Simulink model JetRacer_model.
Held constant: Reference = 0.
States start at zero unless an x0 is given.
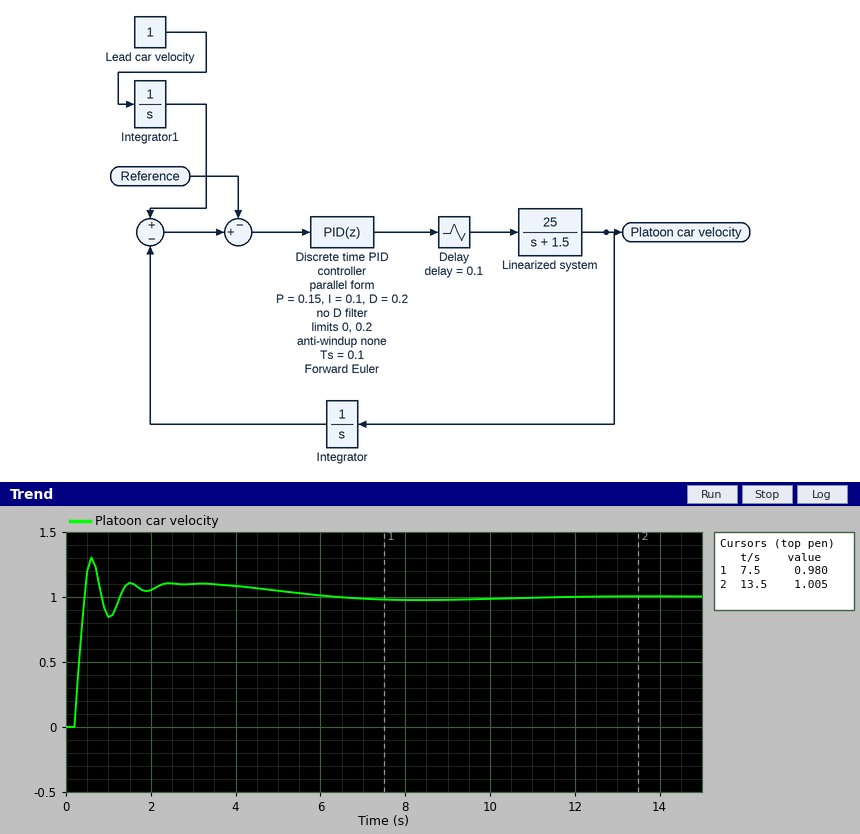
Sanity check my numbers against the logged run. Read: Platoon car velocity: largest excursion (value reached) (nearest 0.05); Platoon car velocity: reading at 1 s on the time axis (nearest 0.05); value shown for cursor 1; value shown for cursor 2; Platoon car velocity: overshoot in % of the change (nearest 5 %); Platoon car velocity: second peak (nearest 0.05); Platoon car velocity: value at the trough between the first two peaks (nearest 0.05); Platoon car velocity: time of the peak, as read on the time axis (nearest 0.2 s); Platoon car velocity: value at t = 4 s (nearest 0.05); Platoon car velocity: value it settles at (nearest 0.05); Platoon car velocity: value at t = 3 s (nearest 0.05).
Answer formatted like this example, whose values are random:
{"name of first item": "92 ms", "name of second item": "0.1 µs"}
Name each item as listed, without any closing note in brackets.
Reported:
{"Platoon car velocity: largest excursion (value reached)": "1.30", "Platoon car velocity: reading at 1 s on the time axis": "0.85", "value shown for cursor 1": "0.980", "value shown for cursor 2": "1.005", "Platoon car velocity: overshoot in % of the change": "30 %", "Platoon car velocity: second peak": "1.10", "Platoon car velocity: value at the trough between the first two peaks": "0.85", "Platoon car velocity: time of the peak, as read on the time axis": "0.6 s", "Platoon car velocity: value at t = 4 s": "1.10", "Platoon car velocity: value it settles at": "1.00", "Platoon car velocity: value at t = 3 s": "1.10"}
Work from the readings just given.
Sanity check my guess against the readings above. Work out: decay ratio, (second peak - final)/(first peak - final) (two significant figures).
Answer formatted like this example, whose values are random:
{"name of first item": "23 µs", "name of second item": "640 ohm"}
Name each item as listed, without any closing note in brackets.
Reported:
{"decay ratio, (second peak - final)/(first peak - final)": "0.33"}
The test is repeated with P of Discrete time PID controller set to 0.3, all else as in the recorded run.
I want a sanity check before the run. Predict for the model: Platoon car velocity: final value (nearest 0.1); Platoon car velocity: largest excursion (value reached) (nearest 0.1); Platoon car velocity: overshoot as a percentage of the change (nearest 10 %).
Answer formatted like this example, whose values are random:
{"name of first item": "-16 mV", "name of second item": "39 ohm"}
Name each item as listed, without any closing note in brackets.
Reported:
{"Platoon car velocity: final value": "1.0", "Platoon car velocity: largest excursion (value reached)": "1.4", "Platoon car velocity: overshoot as a percentage of the change": "40 %"}
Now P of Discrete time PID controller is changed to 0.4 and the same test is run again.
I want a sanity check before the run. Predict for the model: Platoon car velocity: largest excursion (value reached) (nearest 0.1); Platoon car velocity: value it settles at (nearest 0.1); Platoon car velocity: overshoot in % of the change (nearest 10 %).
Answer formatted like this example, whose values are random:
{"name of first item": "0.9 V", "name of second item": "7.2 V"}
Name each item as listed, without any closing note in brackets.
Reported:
{"Platoon car velocity: largest excursion (value reached)": "1.6", "Platoon car velocity: value it settles at": "1.0", "Platoon car velocity: overshoot in % of the change": "60 %"}
